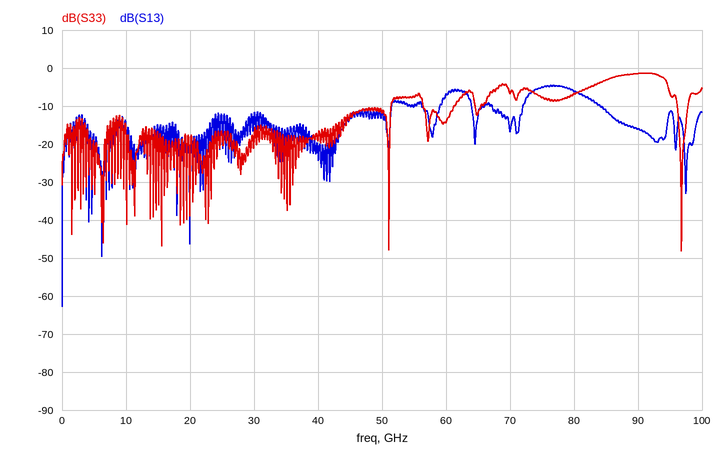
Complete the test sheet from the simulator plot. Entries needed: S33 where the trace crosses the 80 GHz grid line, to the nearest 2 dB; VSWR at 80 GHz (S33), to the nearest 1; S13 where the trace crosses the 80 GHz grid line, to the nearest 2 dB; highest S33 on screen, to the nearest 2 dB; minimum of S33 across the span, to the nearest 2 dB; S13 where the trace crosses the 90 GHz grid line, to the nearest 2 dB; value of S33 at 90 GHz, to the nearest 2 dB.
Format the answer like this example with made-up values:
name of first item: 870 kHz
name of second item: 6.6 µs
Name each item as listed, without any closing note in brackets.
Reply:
S33 where the trace crosses the 80 GHz grid line, to the nearest 2 dB: -6 dB
VSWR at 80 GHz (S33), to the nearest 1: 3
S13 where the trace crosses the 80 GHz grid line, to the nearest 2 dB: -6 dB
highest S33 on screen, to the nearest 2 dB: -2 dB
minimum of S33 across the span, to the nearest 2 dB: -48 dB
S13 where the trace crosses the 90 GHz grid line, to the nearest 2 dB: -16 dB
value of S33 at 90 GHz, to the nearest 2 dB: -2 dB
